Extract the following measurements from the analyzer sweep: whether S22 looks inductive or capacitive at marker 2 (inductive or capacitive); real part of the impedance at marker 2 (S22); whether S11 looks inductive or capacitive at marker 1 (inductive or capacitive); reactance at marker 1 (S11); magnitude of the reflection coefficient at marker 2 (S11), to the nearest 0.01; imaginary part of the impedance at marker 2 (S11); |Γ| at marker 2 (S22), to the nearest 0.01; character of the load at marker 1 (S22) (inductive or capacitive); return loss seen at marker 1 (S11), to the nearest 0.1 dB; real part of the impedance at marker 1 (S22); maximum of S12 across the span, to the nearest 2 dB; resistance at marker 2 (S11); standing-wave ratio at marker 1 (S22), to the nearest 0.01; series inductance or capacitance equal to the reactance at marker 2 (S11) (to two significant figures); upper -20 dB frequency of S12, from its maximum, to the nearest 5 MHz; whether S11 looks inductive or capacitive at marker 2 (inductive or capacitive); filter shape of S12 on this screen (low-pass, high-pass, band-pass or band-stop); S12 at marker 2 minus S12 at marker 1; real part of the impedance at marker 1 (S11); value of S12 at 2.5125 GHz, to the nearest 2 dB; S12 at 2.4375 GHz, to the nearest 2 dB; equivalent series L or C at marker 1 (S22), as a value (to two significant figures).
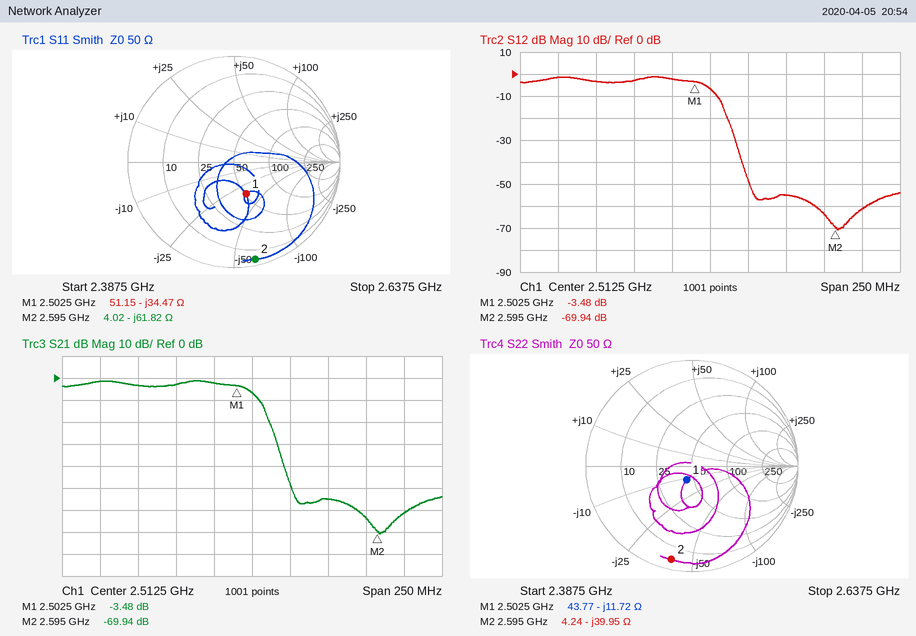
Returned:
capacitive
4.24 Ω
capacitive
-34.47 Ω
0.94
-61.82 Ω
0.90
capacitive
9.8 dB
43.77 Ω
-2 dB
4.02 Ω
1.33
990 fF
2.525 GHz
capacitive
low-pass
-66.46 dB
51.15 Ω
-6 dB
-4 dB
5.4 pF
